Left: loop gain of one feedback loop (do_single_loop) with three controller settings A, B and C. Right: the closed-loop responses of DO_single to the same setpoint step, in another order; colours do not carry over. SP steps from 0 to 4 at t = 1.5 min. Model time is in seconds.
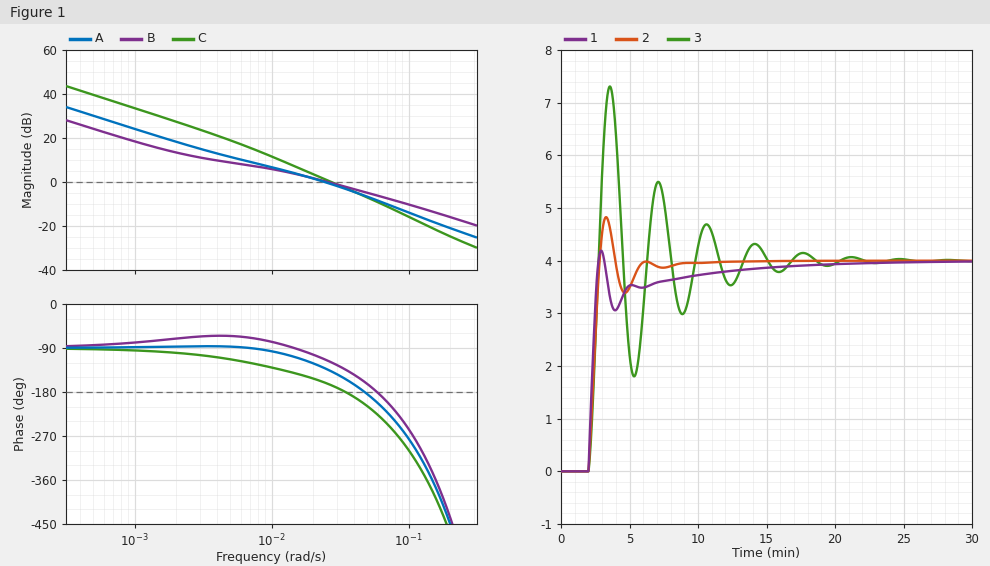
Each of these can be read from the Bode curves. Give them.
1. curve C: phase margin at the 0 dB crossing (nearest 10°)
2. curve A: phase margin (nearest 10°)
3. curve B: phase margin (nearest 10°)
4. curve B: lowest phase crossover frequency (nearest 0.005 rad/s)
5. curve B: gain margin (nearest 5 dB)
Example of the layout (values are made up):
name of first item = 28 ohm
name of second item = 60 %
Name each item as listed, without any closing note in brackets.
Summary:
curve C: phase margin at the 0 dB crossing = 10°
curve A: phase margin = 50°
curve B: phase margin = 60°
curve B: lowest phase crossover frequency = 0.060 rad/s
curve B: gain margin = 5 dB
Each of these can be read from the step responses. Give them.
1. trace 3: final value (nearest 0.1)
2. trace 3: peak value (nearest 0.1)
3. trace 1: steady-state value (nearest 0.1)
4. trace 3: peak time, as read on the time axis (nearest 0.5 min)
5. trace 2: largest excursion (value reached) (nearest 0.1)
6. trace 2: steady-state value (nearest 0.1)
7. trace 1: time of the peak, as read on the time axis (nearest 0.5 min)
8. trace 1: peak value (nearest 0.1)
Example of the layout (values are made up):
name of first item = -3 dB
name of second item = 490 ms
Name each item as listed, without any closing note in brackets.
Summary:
trace 3: final value = 4.0
trace 3: peak value = 7.3
trace 1: steady-state value = 4.0
trace 3: peak time, as read on the time axis = 3.5 min
trace 2: largest excursion (value reached) = 4.8
trace 2: steady-state value = 4.0
trace 1: time of the peak, as read on the time axis = 3.0 min
trace 1: peak value = 4.2
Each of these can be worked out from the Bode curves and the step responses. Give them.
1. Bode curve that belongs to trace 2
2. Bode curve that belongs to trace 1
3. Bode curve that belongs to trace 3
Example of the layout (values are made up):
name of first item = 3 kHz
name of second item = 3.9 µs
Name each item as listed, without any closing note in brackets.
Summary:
Bode curve that belongs to trace 2 = A
Bode curve that belongs to trace 1 = B
Bode curve that belongs to trace 3 = C
